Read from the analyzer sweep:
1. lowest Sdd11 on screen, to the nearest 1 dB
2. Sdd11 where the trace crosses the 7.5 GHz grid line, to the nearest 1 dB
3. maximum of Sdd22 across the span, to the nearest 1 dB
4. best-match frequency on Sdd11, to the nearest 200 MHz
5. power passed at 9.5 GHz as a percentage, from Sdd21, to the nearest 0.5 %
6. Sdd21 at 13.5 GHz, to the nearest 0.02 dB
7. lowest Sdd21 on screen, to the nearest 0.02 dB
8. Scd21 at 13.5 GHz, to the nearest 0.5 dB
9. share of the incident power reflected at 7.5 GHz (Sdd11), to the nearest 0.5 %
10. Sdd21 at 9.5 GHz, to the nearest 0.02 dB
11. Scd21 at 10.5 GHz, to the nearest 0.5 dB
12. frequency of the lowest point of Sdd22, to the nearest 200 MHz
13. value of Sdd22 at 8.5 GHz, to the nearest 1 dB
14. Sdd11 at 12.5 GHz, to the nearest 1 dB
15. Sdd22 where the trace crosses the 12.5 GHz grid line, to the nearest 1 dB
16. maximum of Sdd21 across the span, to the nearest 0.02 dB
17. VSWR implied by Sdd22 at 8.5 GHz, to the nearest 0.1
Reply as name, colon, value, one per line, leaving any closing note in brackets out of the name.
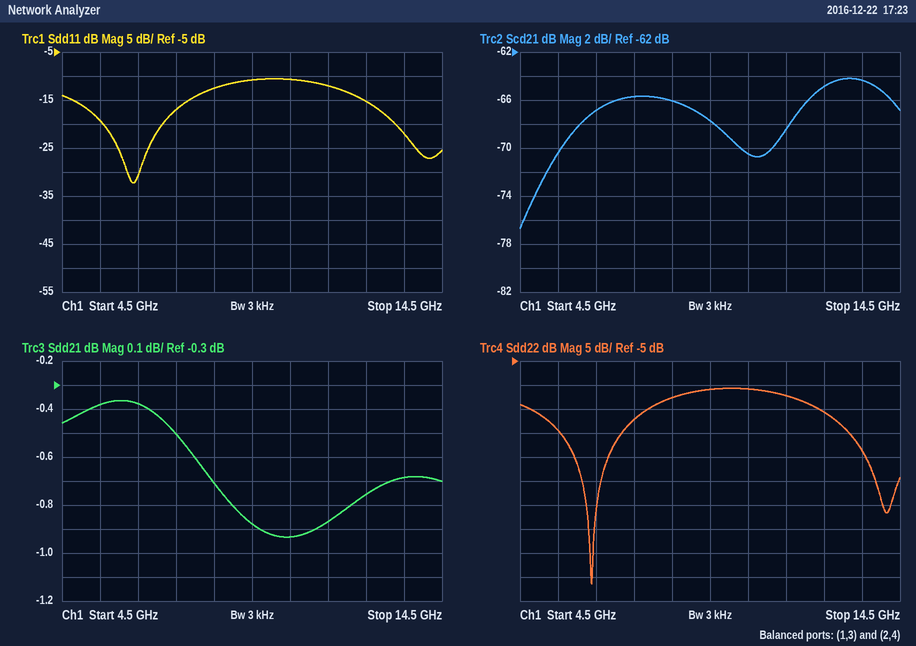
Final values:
lowest Sdd11 on screen, to the nearest 1 dB: -32 dB
Sdd11 where the trace crosses the 7.5 GHz grid line, to the nearest 1 dB: -17 dB
maximum of Sdd22 across the span, to the nearest 1 dB: -11 dB
best-match frequency on Sdd11, to the nearest 200 MHz: 6.4 GHz
power passed at 9.5 GHz as a percentage, from Sdd21, to the nearest 0.5 %: 81.5 %
Sdd21 at 13.5 GHz, to the nearest 0.02 dB: -0.68 dB
lowest Sdd21 on screen, to the nearest 0.02 dB: -0.94 dB
Scd21 at 13.5 GHz, to the nearest 0.5 dB: -64.5 dB
share of the incident power reflected at 7.5 GHz (Sdd11), to the nearest 0.5 %: 2.0 %
Sdd21 at 9.5 GHz, to the nearest 0.02 dB: -0.88 dB
Scd21 at 10.5 GHz, to the nearest 0.5 dB: -70.5 dB
frequency of the lowest point of Sdd22, to the nearest 200 MHz: 6.4 GHz
value of Sdd22 at 8.5 GHz, to the nearest 1 dB: -13 dB
Sdd11 at 12.5 GHz, to the nearest 1 dB: -15 dB
Sdd22 where the trace crosses the 12.5 GHz grid line, to the nearest 1 dB: -16 dB
maximum of Sdd21 across the span, to the nearest 0.02 dB: -0.36 dB
VSWR implied by Sdd22 at 8.5 GHz, to the nearest 0.1: 1.6
